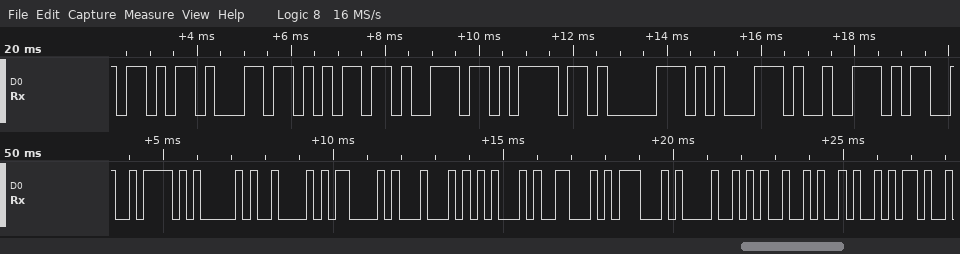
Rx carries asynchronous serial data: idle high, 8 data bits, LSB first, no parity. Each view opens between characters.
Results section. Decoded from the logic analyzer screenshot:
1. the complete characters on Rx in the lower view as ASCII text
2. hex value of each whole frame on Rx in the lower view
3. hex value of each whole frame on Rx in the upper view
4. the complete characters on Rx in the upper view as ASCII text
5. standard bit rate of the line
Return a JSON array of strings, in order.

["\"zABCDEFGHIJ\"", "7A, 41, 42, 43, 44, 45, 46, 47, 48, 49, 4A", "6B, 6C, 6D, 6E, 6F, 70, 71, 72", "\"klmnopqr\"", "4800 baud"]
